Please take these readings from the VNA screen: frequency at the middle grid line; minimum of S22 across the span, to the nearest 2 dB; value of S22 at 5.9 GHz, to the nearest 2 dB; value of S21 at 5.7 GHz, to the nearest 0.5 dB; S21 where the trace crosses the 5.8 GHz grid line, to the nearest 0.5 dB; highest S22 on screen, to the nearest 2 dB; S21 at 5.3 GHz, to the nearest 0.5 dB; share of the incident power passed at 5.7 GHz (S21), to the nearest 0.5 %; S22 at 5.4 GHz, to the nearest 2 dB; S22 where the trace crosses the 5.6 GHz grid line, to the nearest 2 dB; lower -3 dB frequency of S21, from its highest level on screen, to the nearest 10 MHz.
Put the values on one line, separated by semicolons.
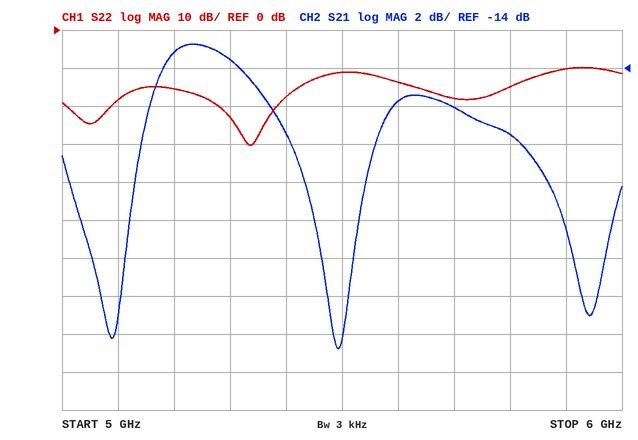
5.5 GHz; -30 dB; -10 dB; -16.0 dB; -17.5 dB; -10 dB; -13.5 dB; 2.5 %; -18 dB; -14 dB; 5.16 GHz
